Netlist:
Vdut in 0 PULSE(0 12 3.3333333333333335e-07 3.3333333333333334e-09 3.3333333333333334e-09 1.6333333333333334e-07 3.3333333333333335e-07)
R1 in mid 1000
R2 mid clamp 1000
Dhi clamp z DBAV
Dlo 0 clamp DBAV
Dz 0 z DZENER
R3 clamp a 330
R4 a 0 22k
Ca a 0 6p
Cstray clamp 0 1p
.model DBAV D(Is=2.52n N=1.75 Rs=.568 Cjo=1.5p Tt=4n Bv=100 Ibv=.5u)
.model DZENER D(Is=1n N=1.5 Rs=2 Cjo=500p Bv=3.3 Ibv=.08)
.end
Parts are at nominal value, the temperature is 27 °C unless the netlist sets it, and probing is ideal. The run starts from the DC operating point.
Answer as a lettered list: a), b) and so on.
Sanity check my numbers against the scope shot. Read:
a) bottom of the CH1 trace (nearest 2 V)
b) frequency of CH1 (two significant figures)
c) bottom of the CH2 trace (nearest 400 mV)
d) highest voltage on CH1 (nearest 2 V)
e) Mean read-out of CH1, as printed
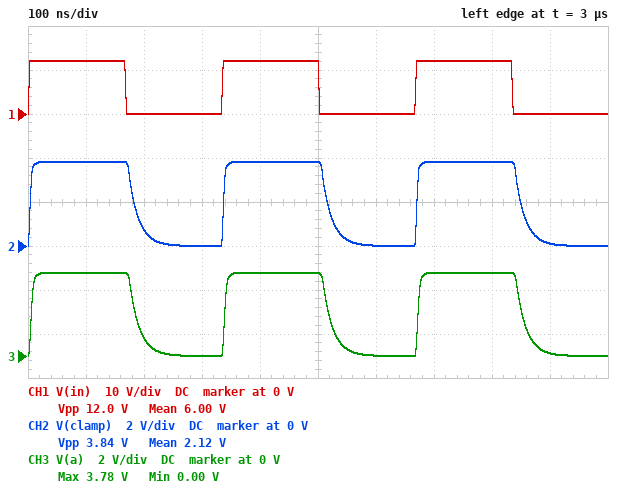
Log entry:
a) 0 V
b) 3.0 MHz
c) 0 V
d) 12 V
e) 6.00 V
